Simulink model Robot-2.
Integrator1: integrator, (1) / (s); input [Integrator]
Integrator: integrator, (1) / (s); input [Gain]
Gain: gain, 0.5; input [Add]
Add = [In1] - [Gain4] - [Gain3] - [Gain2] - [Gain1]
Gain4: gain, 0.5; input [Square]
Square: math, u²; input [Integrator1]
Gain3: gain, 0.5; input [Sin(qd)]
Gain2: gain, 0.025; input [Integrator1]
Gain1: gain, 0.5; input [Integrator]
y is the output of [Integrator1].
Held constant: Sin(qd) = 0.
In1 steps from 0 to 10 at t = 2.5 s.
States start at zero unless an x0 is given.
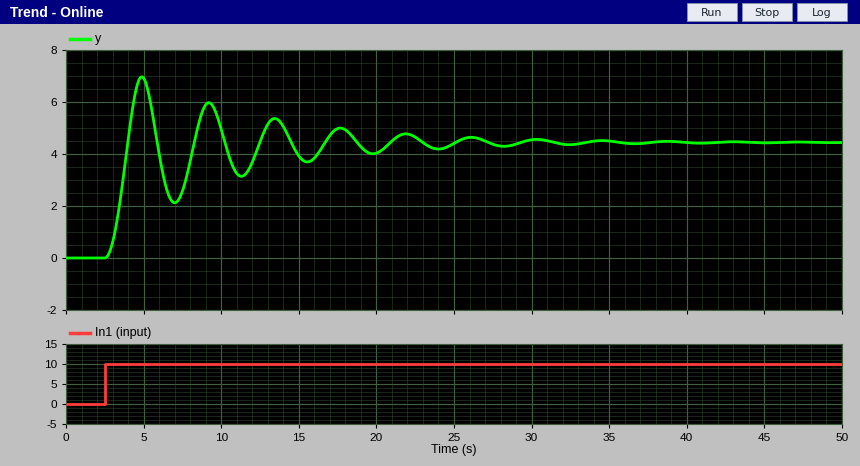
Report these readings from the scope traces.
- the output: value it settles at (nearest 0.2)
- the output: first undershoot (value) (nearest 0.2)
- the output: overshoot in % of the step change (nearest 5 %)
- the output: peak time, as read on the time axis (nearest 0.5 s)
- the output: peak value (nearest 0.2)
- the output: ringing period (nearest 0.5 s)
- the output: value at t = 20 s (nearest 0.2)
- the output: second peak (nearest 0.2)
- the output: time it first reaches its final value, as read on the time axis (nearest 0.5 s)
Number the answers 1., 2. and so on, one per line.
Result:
1. 4.4
2. 2.2
3. 55 %
4. 5.0 s
5. 7.0
6. 4.5 s
7. 4.0
8. 6.0
9. 4.0 s
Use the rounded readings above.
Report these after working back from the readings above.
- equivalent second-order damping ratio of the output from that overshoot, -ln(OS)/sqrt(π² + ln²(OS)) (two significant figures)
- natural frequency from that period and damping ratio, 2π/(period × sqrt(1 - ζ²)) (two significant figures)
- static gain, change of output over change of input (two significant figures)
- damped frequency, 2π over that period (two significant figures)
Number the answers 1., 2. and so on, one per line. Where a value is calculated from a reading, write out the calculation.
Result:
1. ln(0.55) = -0.598; 0.598 / sqrt(9.870 + 0.357) = 0.19
2. 2π / (4.5 × sqrt(1 - 0.19²)) = 1.4 rad/s
3. (4.4 - 0) / (10 - 0) = 0.44
4. 2π / 4.5 = 1.4 rad/s
